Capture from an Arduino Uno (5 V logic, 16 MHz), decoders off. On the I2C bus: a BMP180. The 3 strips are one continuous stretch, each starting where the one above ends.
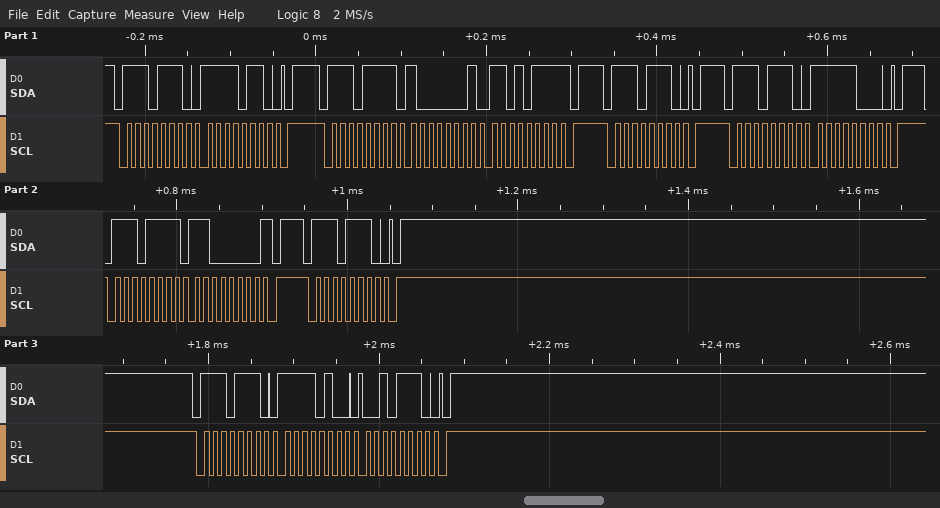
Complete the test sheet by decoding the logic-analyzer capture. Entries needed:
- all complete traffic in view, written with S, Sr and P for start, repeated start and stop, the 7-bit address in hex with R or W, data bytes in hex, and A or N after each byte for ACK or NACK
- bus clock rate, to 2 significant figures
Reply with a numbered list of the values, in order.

1. S 77W A F6 A P S 77R A 81 A D7 N P S 77W A P S 77W A F8 A P S 77R A C0 N P S 77W A P S 77W A F4 A 2E A P
2. 100 kHz
